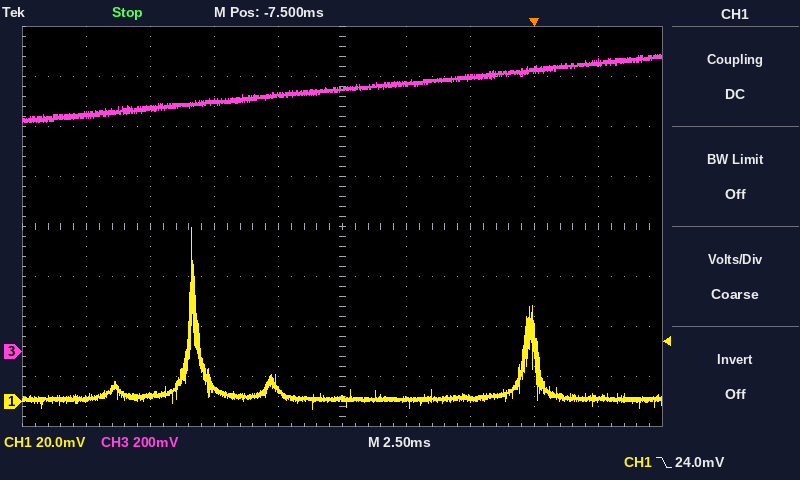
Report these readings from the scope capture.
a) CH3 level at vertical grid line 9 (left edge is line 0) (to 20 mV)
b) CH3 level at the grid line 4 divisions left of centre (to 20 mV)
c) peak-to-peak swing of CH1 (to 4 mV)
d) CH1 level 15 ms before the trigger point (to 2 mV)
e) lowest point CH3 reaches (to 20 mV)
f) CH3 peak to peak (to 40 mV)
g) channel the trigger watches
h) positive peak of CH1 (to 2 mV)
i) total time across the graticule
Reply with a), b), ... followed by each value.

a) 1.16 V
b) 940 mV
c) 72 mV
d) 2 mV
e) 920 mV
f) 280 mV
g) CH1
h) 70 mV
i) 25 ms
